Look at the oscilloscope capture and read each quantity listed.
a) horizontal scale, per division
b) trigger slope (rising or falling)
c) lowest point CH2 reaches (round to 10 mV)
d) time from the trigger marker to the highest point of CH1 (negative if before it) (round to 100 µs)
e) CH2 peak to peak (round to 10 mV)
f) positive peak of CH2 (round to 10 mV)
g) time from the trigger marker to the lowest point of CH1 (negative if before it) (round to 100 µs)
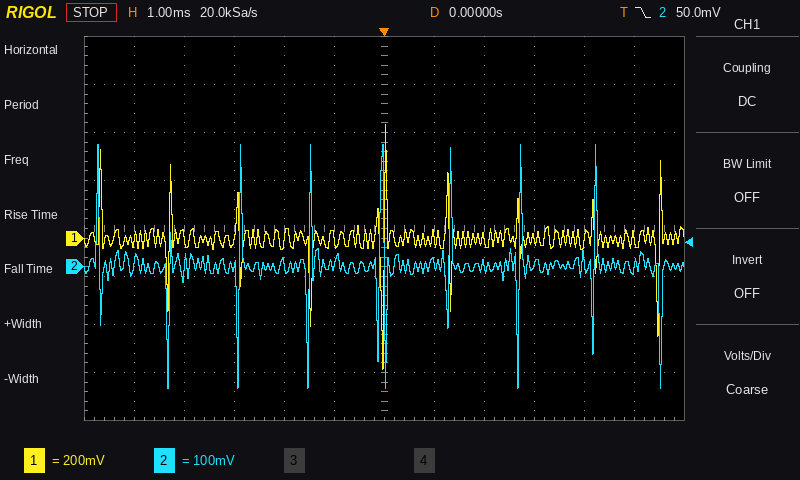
1 ms
falling
-250 mV
0.0 ms
510 mV
260 mV
0.0 ms
